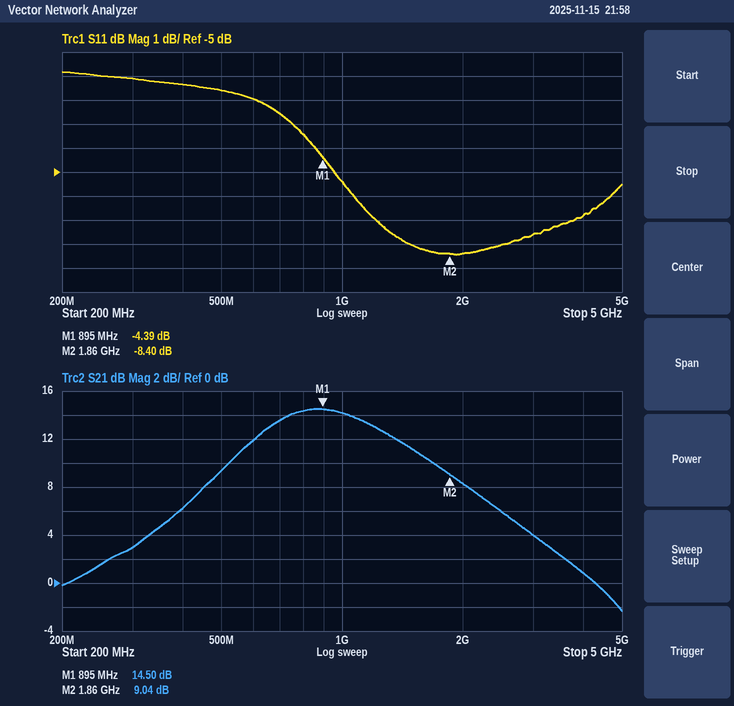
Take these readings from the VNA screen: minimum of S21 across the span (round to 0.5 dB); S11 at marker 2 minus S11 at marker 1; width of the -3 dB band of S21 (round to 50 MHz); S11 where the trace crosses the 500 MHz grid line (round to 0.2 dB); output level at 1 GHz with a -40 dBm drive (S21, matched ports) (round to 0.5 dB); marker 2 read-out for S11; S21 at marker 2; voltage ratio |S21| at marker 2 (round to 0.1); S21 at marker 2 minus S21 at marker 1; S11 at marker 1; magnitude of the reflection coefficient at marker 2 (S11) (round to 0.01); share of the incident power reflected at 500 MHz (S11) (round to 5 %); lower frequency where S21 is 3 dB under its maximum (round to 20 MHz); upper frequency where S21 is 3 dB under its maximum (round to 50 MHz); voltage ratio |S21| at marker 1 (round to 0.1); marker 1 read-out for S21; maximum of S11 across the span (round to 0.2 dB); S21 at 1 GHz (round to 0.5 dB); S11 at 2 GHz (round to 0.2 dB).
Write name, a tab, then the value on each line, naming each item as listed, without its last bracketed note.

minimum of S21 across the span	-2.5 dB
S11 at marker 2 minus S11 at marker 1	-4.01 dB
width of the -3 dB band of S21	850 MHz
S11 where the trace crosses the 500 MHz grid line	-1.6 dB
output level at 1 GHz with a -40 dBm drive (S21, matched ports)	-26.0 dBm
marker 2 read-out for S11	-8.40 dB
S21 at marker 2	9.04 dB
voltage ratio |S21| at marker 2	2.8
S21 at marker 2 minus S21 at marker 1	-5.46 dB
S11 at marker 1	-4.39 dB
magnitude of the reflection coefficient at marker 2 (S11)	0.38
share of the incident power reflected at 500 MHz (S11)	70 %
lower frequency where S21 is 3 dB under its maximum	580 MHz
upper frequency where S21 is 3 dB under its maximum	1.45 GHz
voltage ratio |S21| at marker 1	5.3
marker 1 read-out for S21	14.50 dB
maximum of S11 across the span	-0.8 dB
S21 at 1 GHz	14.0 dB
S11 at 2 GHz	-8.4 dB
